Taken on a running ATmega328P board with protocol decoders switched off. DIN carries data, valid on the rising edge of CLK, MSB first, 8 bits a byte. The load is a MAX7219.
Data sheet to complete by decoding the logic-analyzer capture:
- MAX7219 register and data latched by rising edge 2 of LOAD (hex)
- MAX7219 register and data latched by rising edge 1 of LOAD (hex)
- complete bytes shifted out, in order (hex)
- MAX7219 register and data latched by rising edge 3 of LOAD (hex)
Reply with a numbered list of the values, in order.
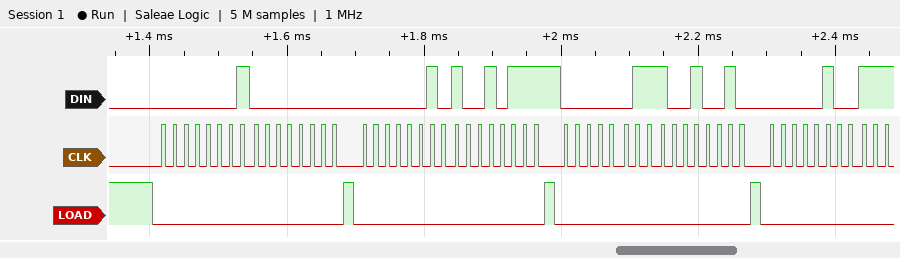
1. register 0x2, data 0x97
2. register 0x1, data 0x00
3. 01 00 02 97 03 92 04
4. register 0x3, data 0x92
